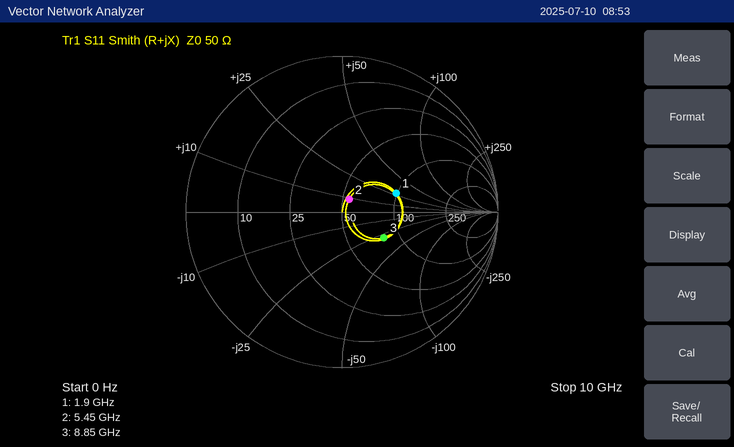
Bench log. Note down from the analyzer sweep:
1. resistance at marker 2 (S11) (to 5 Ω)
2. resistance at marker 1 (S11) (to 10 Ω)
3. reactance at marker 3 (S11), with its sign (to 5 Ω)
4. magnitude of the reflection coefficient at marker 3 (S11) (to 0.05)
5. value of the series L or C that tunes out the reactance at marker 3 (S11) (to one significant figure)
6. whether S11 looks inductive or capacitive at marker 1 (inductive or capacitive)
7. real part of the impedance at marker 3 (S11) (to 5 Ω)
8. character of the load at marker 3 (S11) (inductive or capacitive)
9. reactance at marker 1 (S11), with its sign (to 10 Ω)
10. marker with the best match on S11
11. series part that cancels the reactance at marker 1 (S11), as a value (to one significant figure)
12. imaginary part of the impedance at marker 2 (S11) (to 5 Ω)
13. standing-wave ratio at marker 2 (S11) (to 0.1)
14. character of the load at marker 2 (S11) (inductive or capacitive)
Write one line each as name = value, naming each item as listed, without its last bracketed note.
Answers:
resistance at marker 2 (S11) = 55 Ω
resistance at marker 1 (S11) = 100 Ω
reactance at marker 3 (S11), with its sign = -30 Ω
magnitude of the reflection coefficient at marker 3 (S11) = 0.30
value of the series L or C that tunes out the reactance at marker 3 (S11) = 500 pH
whether S11 looks inductive or capacitive at marker 1 = inductive
real part of the impedance at marker 3 (S11) = 80 Ω
character of the load at marker 3 (S11) = capacitive
reactance at marker 1 (S11), with its sign = +30 Ω
marker with the best match on S11 = marker 2
series part that cancels the reactance at marker 1 (S11), as a value = 3 pF
imaginary part of the impedance at marker 2 (S11) = +10 Ω
standing-wave ratio at marker 2 (S11) = 1.2
character of the load at marker 2 (S11) = inductive
